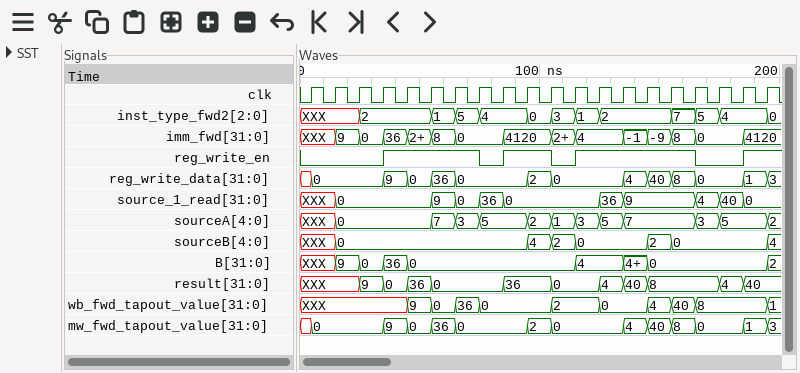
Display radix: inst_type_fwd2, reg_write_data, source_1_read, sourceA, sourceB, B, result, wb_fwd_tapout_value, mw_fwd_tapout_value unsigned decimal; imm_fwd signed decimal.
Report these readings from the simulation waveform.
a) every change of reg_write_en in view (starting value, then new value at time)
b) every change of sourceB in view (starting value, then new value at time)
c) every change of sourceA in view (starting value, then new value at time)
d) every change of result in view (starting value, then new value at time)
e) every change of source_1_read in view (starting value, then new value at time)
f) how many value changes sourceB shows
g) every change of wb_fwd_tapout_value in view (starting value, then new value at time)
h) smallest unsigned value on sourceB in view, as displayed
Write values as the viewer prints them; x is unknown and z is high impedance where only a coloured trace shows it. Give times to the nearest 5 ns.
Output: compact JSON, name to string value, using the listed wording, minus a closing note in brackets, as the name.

{"every change of reg_write_en in view": "0, 1 at 35 ns, 0 at 75 ns, 1 at 85 ns, 0 at 105 ns, 1 at 115 ns, 0 at 165 ns, 1 at 185 ns", "every change of sourceB in view": "XXX, 0 at 15 ns, 4 at 95 ns, 2 at 105 ns, 0 at 115 ns, 2 at 145 ns, 0 at 155 ns, 4 at 195 ns", "every change of sourceA in view": "XXX, 0 at 15 ns, 7 at 55 ns, 3 at 65 ns, 5 at 75 ns, 2 at 95 ns, 1 at 105 ns, 3 at 115 ns, 5 at 125 ns, 7 at 135 ns, 3 at 165 ns, 5 at 175 ns, 2 at 195 ns", "every change of result in view": "XXX, 9 at 25 ns, 0 at 35 ns, 36 at 45 ns, 0 at 55 ns, 36 at 85 ns, 0 at 105 ns, 4 at 125 ns, 40 at 135 ns, 8 at 145 ns, 4 at 175 ns, 40 at 185 ns", "every change of source_1_read in view": "XXX, 0 at 15 ns, 9 at 55 ns, 0 at 65 ns, 36 at 75 ns, 0 at 85 ns, 36 at 125 ns, 9 at 135 ns, 4 at 165 ns, 40 at 175 ns, 0 at 185 ns", "how many value changes sourceB shows": "7", "every change of wb_fwd_tapout_value in view": "XXX, 9 at 45 ns, 0 at 55 ns, 36 at 65 ns, 0 at 75 ns, 2 at 105 ns, 0 at 125 ns, 4 at 145 ns, 40 at 155 ns, 8 at 165 ns, 1 at 195 ns", "smallest unsigned value on sourceB in view, as displayed": "0"}
